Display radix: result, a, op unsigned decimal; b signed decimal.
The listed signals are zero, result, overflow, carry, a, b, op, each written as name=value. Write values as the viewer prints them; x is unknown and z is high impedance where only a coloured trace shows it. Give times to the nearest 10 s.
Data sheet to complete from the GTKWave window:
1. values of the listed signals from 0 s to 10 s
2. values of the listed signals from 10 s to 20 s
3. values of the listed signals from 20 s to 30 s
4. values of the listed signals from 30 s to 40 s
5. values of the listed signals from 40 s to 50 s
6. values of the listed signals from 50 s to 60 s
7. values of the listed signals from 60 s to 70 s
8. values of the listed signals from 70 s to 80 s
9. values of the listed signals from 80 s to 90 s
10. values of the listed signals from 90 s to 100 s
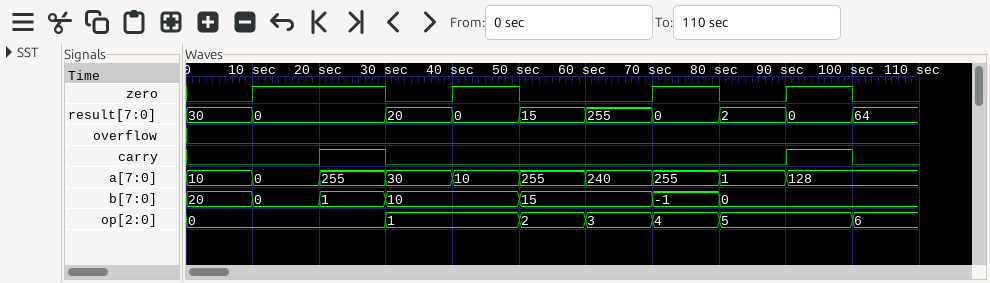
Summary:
zero=0, result=30, overflow=0, carry=0, a=10, b=20, op=0
zero=1, result=0, overflow=0, carry=0, a=0, b=0, op=0
zero=1, result=0, overflow=0, carry=1, a=255, b=1, op=0
zero=0, result=20, overflow=0, carry=0, a=30, b=10, op=1
zero=1, result=0, overflow=0, carry=0, a=10, b=10, op=1
zero=0, result=15, overflow=0, carry=0, a=255, b=15, op=2
zero=0, result=255, overflow=0, carry=0, a=240, b=15, op=3
zero=1, result=0, overflow=0, carry=0, a=255, b=-1, op=4
zero=0, result=2, overflow=0, carry=0, a=1, b=0, op=5
zero=1, result=0, overflow=0, carry=1, a=128, b=0, op=5
